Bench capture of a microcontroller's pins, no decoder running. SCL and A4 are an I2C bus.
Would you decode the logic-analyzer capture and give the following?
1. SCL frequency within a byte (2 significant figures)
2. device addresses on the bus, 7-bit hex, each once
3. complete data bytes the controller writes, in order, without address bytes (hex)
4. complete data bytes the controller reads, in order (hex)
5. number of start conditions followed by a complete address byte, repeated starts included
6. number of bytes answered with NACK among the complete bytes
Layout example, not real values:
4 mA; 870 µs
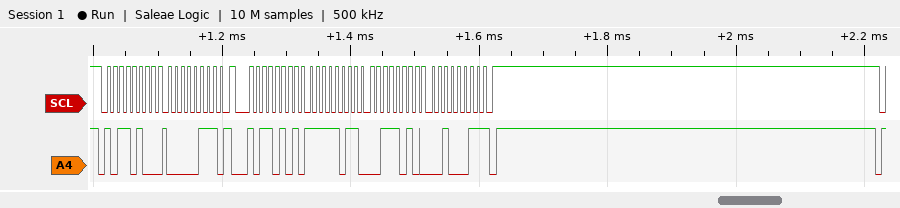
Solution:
100 kHz; 0x5A; 07; FB 3A 23; 2; 1
